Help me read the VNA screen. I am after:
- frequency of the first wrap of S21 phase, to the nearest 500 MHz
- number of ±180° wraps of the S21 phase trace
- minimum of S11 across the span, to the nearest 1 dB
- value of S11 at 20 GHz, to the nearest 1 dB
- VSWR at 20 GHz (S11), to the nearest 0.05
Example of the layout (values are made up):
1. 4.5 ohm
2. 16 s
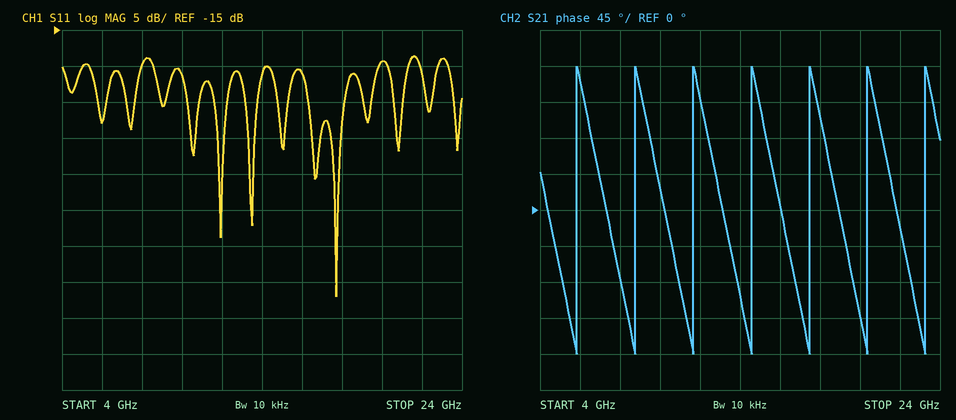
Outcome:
1. 6.0 GHz
2. 7
3. -52 dB
4. -19 dB
5. 1.25
